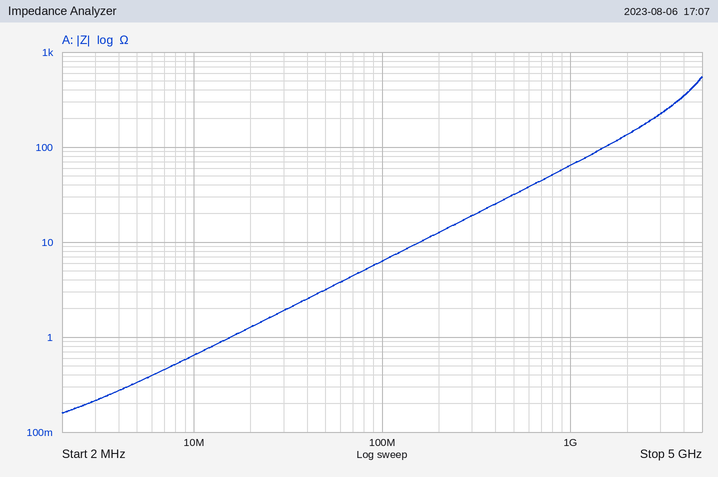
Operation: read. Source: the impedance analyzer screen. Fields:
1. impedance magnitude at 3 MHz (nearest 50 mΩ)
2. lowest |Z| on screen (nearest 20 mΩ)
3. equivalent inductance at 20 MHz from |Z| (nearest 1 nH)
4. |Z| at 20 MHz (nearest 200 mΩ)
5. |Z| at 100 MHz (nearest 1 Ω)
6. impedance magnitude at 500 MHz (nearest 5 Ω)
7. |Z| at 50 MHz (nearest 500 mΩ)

200 mΩ
160 mΩ
10 nH
1.2 Ω
6 Ω
30 Ω
3.0 Ω
